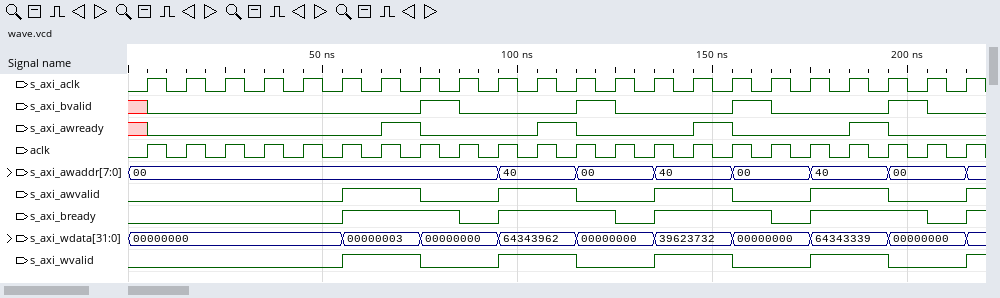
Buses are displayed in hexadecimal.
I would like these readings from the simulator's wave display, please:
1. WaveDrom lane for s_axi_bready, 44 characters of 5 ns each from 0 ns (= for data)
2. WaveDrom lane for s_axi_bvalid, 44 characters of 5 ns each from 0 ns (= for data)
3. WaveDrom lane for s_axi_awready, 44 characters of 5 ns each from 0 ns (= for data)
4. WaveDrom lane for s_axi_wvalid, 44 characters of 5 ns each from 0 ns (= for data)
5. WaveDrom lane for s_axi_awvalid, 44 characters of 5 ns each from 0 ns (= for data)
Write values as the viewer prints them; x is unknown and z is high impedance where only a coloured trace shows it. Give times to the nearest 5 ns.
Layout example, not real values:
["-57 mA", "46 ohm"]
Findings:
["{name: 's_axi_bready', wave: '0..........1.....0.1.....0.1.....0.1.....0.1'}", "{name: 's_axi_bvalid', wave: 'x0.............1.0.....1.0.....1.0.....1.0..'}", "{name: 's_axi_awready', wave: 'x0...........1.0.....1.0.....1.0.....1.0....'}", "{name: 's_axi_wvalid', wave: '0..........1...0...1...0...1...0...1...0...1'}", "{name: 's_axi_awvalid', wave: '0..........1...0...1...0...1...0...1...0...1'}"]
